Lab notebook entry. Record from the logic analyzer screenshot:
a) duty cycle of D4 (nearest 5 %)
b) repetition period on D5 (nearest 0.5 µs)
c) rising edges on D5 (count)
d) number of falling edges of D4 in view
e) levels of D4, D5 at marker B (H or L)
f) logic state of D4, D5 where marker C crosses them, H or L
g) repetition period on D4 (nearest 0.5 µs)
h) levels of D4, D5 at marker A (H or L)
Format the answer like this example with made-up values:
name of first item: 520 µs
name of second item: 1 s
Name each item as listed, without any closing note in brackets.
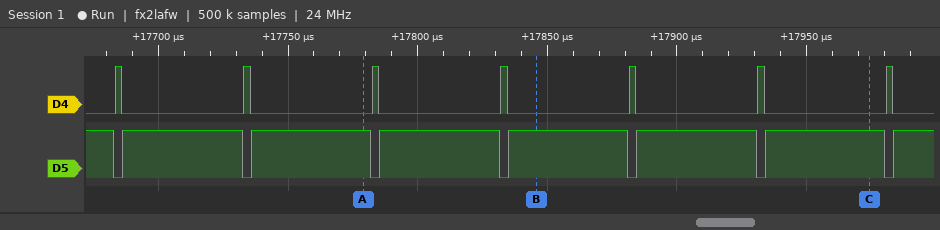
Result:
duty cycle of D4: 5 %
repetition period on D5: 49.5 µs
rising edges on D5: 7
number of falling edges of D4 in view: 7
levels of D4, D5 at marker B: D4=L, D5=H
logic state of D4, D5 where marker C crosses them, H or L: D4=L, D5=H
repetition period on D4: 49.5 µs
levels of D4, D5 at marker A: D4=L, D5=H
